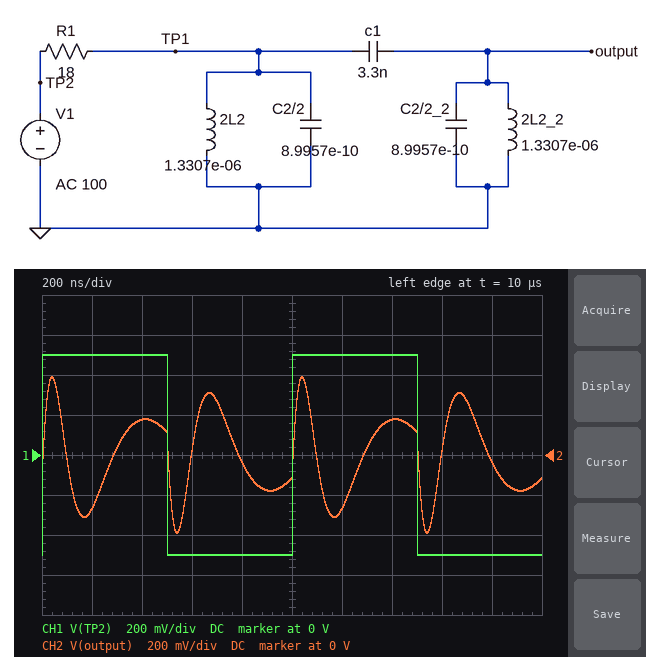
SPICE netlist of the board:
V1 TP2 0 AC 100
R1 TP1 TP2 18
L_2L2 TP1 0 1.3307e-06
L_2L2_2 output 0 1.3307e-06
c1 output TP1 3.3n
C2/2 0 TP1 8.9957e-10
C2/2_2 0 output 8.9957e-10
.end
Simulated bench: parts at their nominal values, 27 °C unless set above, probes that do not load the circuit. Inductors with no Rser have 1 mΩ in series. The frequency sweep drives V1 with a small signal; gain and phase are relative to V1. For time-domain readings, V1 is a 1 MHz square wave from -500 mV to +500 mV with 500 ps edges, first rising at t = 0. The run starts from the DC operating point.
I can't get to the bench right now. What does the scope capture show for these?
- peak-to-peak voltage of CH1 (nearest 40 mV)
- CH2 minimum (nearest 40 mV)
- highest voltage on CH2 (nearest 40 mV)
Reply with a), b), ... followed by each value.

a) 1.00 V
b) -400 mV
c) 400 mV
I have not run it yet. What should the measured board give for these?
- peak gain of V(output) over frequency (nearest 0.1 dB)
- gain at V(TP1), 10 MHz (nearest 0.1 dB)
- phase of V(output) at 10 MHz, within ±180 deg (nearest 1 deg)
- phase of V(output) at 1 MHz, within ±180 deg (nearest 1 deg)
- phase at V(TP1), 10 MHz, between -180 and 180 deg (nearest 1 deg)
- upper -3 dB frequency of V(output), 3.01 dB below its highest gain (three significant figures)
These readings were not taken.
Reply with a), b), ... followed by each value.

a) 3.0 dB
b) -5.0 dB
c) -56 deg
d) -122 deg
e) -56 deg
f) 4.59 MHz
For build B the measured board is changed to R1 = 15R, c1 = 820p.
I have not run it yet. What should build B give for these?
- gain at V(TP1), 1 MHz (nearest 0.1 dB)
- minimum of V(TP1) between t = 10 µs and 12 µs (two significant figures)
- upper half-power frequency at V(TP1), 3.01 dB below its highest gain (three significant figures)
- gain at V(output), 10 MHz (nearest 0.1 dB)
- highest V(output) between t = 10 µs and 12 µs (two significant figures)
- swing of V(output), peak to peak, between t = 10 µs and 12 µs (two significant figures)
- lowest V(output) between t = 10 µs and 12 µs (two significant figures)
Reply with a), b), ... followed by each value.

a) -5.6 dB
b) -680 mV
c) 9.82 MHz
d) -8.5 dB
e) 500 mV
f) 1.0 V
g) -500 mV
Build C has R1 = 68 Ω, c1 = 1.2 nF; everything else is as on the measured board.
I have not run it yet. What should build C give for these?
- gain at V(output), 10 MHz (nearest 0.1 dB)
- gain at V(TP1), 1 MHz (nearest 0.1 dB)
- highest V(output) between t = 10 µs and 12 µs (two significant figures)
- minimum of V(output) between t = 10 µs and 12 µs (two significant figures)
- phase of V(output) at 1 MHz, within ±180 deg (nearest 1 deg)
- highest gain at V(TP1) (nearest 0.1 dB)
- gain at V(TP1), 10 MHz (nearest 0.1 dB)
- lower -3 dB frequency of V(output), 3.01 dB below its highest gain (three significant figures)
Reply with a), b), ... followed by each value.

a) -18.1 dB
b) -17.2 dB
c) 240 mV
d) -240 mV
e) -98 deg
f) 0 dB
g) -14.0 dB
h) 2.32 MHz
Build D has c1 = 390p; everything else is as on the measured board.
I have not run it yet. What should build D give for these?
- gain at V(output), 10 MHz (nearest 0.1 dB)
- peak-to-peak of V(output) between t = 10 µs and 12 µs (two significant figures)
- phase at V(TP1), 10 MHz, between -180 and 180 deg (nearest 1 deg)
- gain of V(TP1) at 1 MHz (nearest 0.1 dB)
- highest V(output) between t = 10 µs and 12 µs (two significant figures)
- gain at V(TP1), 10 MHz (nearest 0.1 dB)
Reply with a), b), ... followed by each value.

a) -12.4 dB
b) 330 mV
c) -47 deg
d) -7.0 dB
e) 170 mV
f) -3.4 dB
